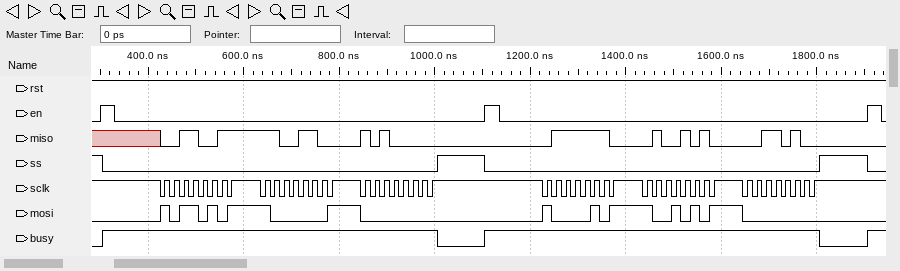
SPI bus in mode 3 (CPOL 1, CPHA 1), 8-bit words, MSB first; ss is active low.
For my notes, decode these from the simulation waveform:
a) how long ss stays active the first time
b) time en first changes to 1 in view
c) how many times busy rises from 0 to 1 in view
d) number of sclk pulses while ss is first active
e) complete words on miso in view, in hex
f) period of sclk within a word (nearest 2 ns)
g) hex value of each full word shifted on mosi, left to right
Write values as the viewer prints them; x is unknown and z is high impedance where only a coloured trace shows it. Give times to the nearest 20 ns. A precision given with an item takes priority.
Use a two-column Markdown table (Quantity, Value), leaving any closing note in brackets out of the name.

| Quantity | Value |
|---|---|
| how long ss stays active the first time | 700 ns |
| time en first changes to 1 in view | 300 ns |
| how many times busy rises from 0 to 1 in view | 3 |
| number of sclk pulses while ss is first active | 24 |
| complete words on miso in view, in hex | 33, CC, A0, 7E, 4A, 34 |
| period of sclk within a word | 20 ns |
| hex value of each full word shifted on mosi, left to right | B5, 81, 00, 85, 95, 00 |
